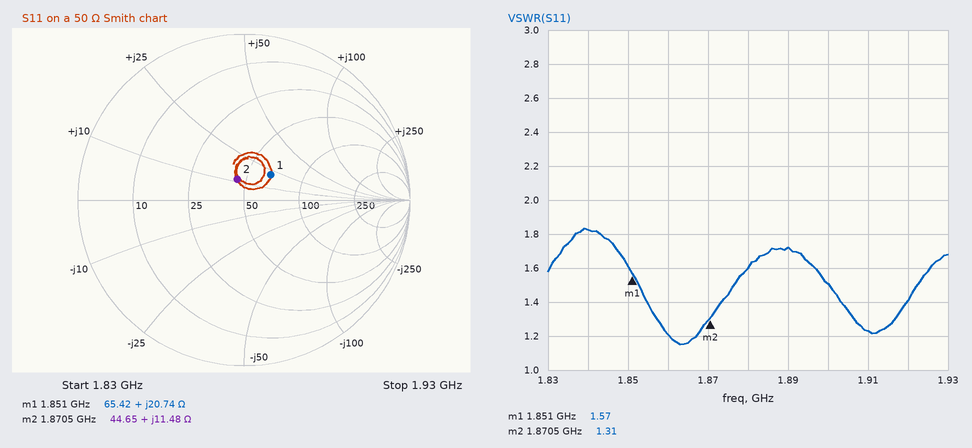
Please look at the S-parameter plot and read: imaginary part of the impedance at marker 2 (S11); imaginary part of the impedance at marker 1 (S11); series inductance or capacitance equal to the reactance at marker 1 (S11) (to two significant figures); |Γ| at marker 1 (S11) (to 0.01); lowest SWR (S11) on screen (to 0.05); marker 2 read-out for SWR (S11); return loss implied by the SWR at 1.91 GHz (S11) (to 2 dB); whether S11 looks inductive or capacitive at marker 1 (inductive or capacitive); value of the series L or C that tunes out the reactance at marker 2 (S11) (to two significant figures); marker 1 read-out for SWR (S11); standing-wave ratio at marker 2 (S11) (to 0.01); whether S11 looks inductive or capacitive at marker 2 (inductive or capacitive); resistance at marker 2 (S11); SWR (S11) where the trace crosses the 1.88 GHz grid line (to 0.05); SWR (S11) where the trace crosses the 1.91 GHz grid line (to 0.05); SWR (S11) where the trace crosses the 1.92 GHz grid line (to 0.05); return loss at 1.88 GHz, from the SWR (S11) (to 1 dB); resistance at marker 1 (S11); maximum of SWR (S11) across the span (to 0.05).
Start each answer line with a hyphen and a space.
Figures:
- +11.48 Ω
- +20.74 Ω
- 1.8 nH
- 0.22
- 1.15
- 1.31
- 20 dB
- inductive
- 7.4 pF
- 1.57
- 1.31
- inductive
- 44.65 Ω
- 1.60
- 1.25
- 1.40
- 13 dB
- 65.42 Ω
- 1.85
